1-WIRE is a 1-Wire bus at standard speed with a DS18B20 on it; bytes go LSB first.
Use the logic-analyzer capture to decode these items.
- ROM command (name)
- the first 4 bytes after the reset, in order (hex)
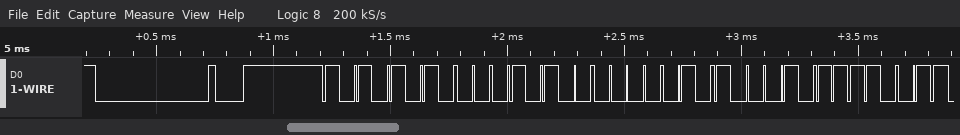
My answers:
Match ROM
55 28 A0 E8
